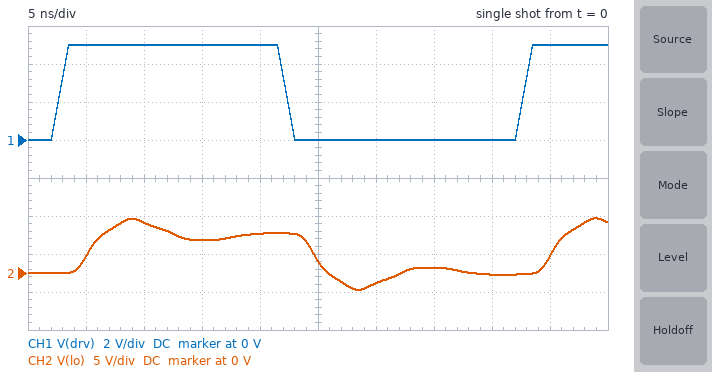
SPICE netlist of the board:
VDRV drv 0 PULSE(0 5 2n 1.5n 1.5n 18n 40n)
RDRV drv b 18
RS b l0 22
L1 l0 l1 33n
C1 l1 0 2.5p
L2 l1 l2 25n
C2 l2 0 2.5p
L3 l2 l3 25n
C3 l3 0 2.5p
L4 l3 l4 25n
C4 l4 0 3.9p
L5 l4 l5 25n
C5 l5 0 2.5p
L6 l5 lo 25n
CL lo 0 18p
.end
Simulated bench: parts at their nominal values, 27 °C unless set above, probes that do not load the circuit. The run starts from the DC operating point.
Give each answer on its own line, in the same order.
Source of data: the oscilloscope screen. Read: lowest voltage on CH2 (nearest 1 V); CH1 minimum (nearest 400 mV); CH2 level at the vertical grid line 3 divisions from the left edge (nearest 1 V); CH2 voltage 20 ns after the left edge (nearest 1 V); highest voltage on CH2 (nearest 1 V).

-2 V
0 V
4 V
5 V
7 V
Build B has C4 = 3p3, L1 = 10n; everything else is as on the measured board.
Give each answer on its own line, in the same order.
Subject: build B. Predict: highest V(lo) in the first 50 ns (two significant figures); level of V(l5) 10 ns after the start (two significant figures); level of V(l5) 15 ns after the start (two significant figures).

6.9 V
6.1 V
4.6 V
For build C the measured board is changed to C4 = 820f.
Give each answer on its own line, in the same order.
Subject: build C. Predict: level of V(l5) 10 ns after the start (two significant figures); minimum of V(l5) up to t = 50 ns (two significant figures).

6.5 V
-1.9 V
